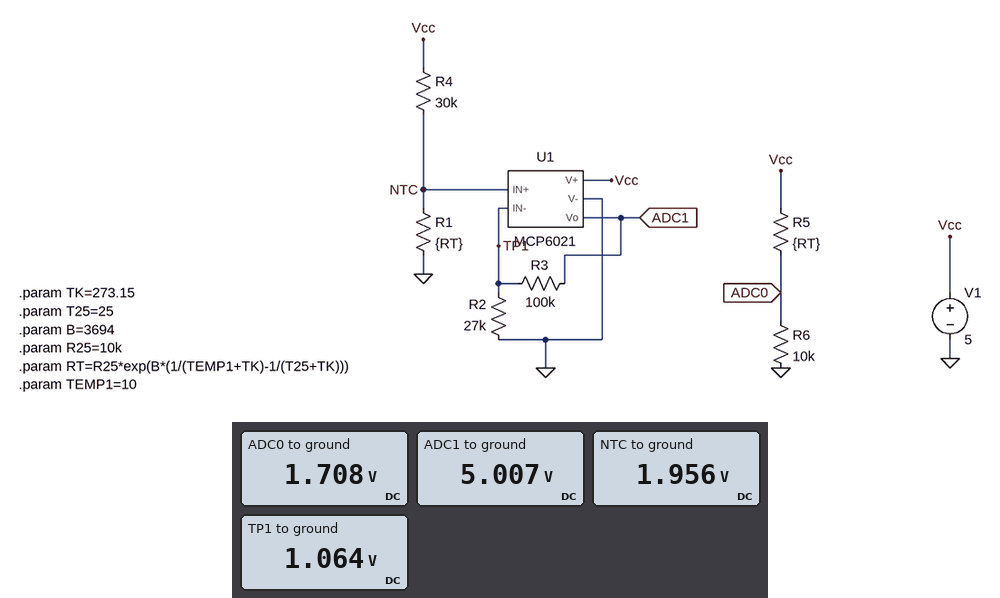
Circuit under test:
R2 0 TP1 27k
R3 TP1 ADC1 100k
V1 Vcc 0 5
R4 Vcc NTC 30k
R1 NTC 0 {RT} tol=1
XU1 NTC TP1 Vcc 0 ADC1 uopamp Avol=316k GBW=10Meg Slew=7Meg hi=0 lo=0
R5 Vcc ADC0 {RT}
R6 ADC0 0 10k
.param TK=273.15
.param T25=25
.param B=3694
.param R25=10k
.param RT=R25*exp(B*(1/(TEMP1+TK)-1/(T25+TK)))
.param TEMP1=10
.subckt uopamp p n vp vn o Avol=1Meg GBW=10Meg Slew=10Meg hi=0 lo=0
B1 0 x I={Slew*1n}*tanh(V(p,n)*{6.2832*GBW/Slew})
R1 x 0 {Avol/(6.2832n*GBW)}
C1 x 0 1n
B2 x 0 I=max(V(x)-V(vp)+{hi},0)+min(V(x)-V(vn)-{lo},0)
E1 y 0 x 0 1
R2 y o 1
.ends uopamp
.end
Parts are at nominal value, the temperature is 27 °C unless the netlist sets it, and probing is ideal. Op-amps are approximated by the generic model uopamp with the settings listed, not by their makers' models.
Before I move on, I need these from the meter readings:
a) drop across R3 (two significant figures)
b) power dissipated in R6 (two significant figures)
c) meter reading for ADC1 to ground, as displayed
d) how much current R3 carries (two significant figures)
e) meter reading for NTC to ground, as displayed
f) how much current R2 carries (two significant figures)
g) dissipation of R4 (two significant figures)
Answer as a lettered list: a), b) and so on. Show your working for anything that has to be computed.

a) 5.007 V - 1.064 V = 3.9 V
b) (1.708 V)^2 / 10 kΩ = 290 µW
c) 5.007 V
d) (5.007 V - 1.064 V) / 100 kΩ = 39 µA
e) 1.956 V
f) (1.064 V) / 27 kΩ = 39 µA
g) (5 V - 1.956 V)^2 / 30 kΩ = 310 µW
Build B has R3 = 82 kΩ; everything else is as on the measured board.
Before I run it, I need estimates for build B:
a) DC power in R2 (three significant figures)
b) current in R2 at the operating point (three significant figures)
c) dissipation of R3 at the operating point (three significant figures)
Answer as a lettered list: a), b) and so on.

a) 57.0 µW
b) 45.9 µA
c) 173 µW
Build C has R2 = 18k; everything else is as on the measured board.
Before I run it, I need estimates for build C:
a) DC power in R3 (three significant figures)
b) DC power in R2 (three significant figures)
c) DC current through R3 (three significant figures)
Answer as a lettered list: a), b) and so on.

a) 180 µW
b) 32.4 µW
c) 42.4 µA
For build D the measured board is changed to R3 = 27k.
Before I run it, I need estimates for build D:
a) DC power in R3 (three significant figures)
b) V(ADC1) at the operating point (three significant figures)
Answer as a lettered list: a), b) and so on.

a) 142 µW
b) 3.91 V
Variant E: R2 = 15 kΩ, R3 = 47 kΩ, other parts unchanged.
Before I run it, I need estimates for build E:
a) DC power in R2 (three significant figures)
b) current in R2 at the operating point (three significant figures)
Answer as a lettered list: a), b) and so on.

a) 97.8 µW
b) 80.8 µA
